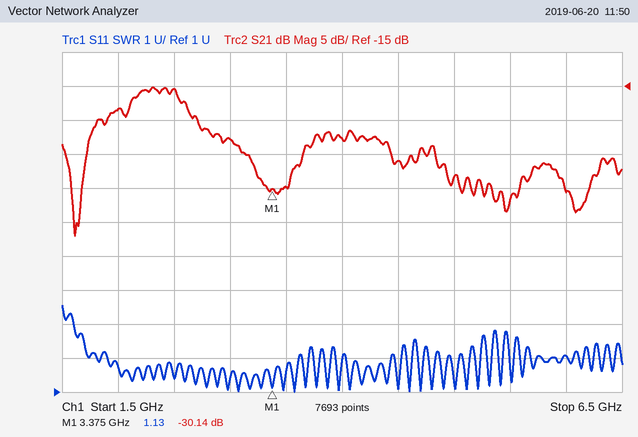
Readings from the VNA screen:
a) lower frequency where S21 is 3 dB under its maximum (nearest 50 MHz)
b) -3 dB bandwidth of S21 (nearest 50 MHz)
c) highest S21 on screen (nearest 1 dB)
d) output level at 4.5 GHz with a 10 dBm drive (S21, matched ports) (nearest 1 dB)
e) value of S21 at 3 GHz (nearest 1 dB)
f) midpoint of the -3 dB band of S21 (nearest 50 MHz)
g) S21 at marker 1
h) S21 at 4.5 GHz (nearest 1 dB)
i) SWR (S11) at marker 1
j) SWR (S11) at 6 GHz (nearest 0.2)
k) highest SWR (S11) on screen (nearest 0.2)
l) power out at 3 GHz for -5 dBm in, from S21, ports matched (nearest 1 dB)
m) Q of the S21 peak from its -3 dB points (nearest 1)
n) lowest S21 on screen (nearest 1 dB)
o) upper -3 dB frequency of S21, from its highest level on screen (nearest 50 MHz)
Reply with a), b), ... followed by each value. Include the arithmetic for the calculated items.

a) 2.10 GHz
b) 2.60 GHz − 2.10 GHz = 500 MHz
c) -15 dB
d) 10 dBm + (-26 dB) = -16 dBm
e) -23 dB
f) 2.35 GHz
g) -30.14 dB
h) -26 dB
i) 1.13
j) 2.0
k) 3.6
l) -5 dBm + (-23 dB) = -28 dBm
m) 2.35 GHz / 500 MHz ≈ 5
n) -37 dB
o) 2.60 GHz
